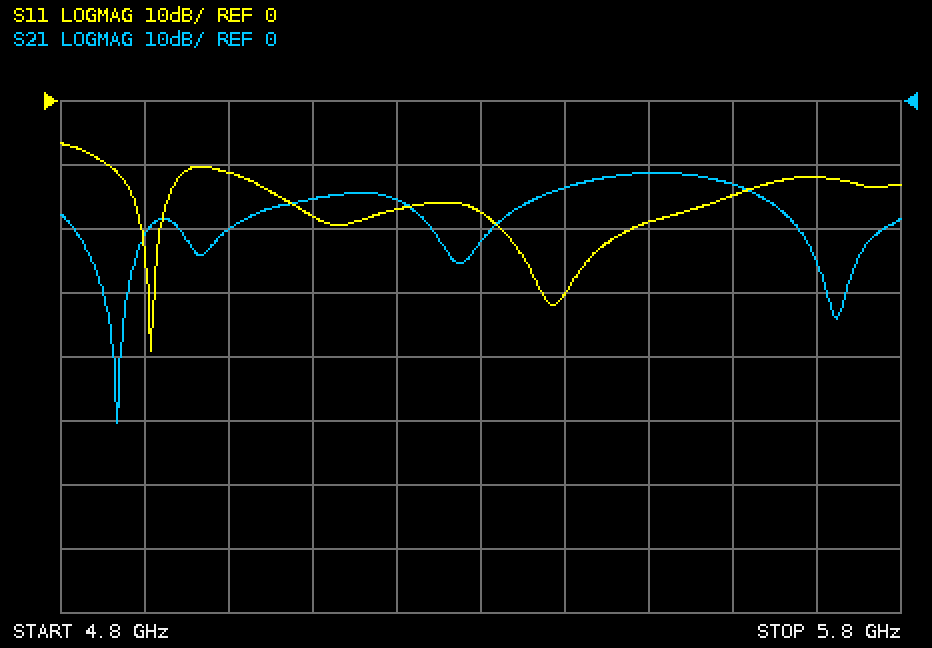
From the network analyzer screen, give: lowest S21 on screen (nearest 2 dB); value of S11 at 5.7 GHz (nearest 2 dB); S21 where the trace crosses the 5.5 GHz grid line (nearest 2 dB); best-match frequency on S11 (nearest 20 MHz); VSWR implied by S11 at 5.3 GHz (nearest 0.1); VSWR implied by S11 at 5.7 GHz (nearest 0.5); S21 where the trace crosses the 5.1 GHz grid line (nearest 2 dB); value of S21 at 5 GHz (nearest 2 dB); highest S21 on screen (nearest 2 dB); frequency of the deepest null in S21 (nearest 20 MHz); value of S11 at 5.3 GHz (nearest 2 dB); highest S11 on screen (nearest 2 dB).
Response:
-50 dB
-12 dB
-12 dB
4.90 GHz
1.3
1.5
-16 dB
-20 dB
-12 dB
4.86 GHz
-18 dB
-6 dB
